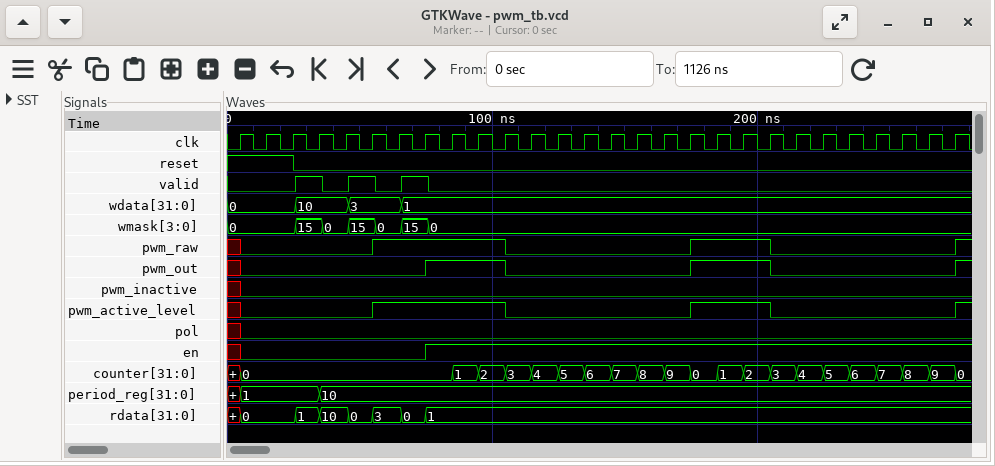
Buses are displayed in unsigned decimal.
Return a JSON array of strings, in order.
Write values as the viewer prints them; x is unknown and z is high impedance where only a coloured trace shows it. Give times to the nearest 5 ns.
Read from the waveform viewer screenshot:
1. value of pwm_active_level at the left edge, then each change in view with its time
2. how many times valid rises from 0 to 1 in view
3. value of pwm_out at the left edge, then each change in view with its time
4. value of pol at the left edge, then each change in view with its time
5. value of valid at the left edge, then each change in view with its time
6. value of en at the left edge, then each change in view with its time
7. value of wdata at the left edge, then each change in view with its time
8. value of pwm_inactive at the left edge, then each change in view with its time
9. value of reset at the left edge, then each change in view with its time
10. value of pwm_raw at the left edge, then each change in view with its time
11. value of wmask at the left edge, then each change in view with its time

["x, 0 at 5 ns, 1 at 55 ns, 0 at 105 ns, 1 at 175 ns, 0 at 205 ns, 1 at 275 ns", "3", "x, 0 at 5 ns, 1 at 75 ns, 0 at 105 ns, 1 at 175 ns, 0 at 205 ns, 1 at 275 ns", "x, 0 at 5 ns", "0, 1 at 25 ns, 0 at 35 ns, 1 at 45 ns, 0 at 55 ns, 1 at 65 ns, 0 at 75 ns", "x, 0 at 5 ns, 1 at 75 ns", "0, 10 at 25 ns, 3 at 45 ns, 1 at 65 ns", "x, 0 at 5 ns", "1, 0 at 25 ns", "x, 0 at 5 ns, 1 at 55 ns, 0 at 105 ns, 1 at 175 ns, 0 at 205 ns, 1 at 275 ns", "0, 15 at 25 ns, 0 at 35 ns, 15 at 45 ns, 0 at 55 ns, 15 at 65 ns, 0 at 75 ns"]
